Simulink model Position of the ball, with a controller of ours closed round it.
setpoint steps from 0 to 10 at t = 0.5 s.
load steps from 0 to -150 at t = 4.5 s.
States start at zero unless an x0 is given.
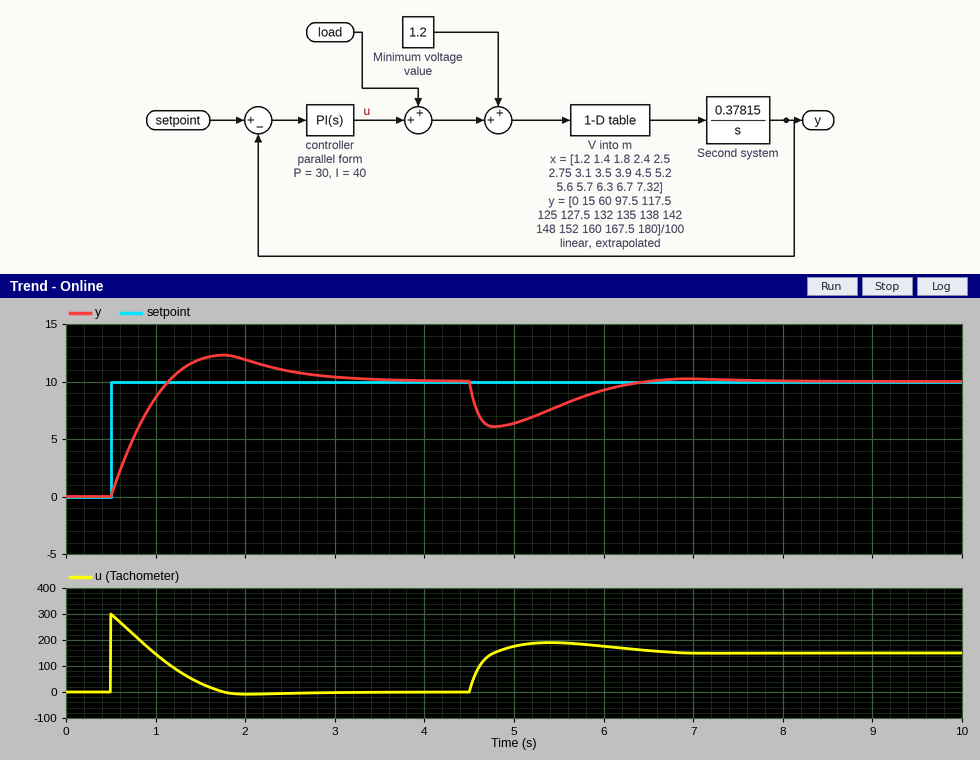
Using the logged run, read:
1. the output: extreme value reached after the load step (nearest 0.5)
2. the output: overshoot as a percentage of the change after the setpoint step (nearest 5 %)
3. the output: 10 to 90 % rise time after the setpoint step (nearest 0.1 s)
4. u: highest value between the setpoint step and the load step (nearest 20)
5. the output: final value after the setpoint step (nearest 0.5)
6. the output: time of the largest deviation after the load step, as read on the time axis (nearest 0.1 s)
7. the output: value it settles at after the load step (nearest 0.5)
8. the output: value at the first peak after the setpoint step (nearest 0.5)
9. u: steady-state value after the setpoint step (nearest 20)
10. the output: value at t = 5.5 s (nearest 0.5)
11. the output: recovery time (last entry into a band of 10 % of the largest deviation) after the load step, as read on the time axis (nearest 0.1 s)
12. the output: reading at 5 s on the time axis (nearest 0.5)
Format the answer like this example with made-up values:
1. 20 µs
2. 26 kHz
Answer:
1. 6.0
2. 25 %
3. 0.5 s
4. 300
5. 10.0
6. 4.8 s
7. 10.0
8. 12.5
9. 0
10. 8.0
11. 6.2 s
12. 6.5
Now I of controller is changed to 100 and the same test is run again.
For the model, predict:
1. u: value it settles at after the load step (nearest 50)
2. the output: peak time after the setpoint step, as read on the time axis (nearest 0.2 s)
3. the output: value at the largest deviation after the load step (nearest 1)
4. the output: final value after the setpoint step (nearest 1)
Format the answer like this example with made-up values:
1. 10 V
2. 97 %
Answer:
1. 150
2. 1.4 s
3. 7
4. 10
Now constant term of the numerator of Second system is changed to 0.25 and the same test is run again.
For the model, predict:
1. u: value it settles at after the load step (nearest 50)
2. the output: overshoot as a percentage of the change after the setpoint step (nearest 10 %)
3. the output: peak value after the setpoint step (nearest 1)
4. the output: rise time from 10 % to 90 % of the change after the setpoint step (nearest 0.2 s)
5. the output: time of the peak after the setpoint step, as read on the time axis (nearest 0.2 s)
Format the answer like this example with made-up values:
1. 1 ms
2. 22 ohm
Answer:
1. 150
2. 30 %
3. 13
4. 0.6 s
5. 2.2 s
